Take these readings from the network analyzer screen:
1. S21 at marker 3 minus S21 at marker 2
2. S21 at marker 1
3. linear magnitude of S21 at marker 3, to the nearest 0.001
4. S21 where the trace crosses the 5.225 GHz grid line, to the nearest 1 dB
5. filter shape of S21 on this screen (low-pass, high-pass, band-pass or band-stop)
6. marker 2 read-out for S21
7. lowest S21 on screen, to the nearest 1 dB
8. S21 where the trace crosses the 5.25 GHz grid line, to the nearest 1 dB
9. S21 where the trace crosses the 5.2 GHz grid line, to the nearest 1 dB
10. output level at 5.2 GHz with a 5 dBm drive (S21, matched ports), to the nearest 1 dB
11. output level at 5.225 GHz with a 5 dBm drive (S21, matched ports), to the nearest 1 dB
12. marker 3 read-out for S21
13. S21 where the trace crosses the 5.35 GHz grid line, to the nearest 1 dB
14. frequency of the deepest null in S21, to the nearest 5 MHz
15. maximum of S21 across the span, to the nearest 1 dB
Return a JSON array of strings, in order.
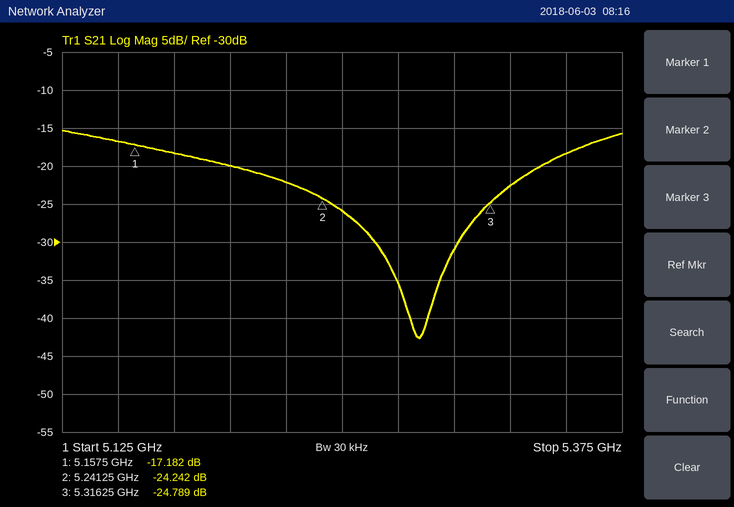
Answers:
["-0.547 dB", "-17.182 dB", "0.058", "-22 dB", "band-stop", "-24.242 dB", "-43 dB", "-26 dB", "-20 dB", "-15 dBm", "-17 dBm", "-24.789 dB", "-18 dB", "5.285 GHz", "-15 dB"]
